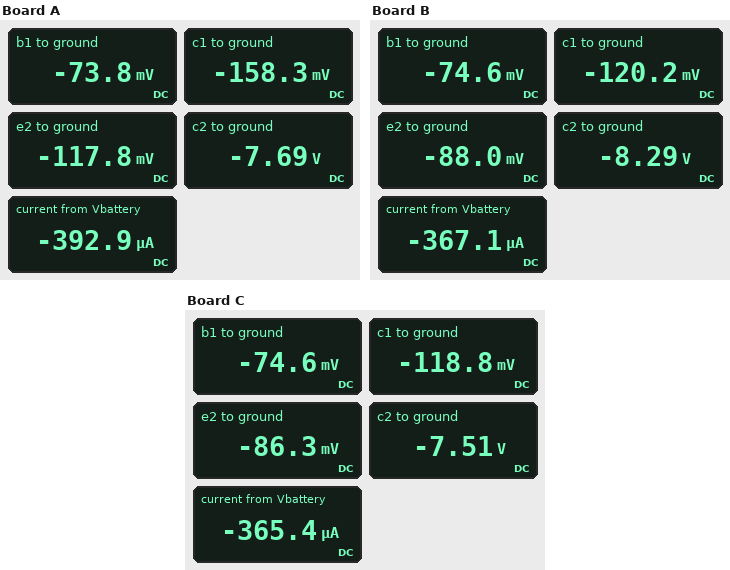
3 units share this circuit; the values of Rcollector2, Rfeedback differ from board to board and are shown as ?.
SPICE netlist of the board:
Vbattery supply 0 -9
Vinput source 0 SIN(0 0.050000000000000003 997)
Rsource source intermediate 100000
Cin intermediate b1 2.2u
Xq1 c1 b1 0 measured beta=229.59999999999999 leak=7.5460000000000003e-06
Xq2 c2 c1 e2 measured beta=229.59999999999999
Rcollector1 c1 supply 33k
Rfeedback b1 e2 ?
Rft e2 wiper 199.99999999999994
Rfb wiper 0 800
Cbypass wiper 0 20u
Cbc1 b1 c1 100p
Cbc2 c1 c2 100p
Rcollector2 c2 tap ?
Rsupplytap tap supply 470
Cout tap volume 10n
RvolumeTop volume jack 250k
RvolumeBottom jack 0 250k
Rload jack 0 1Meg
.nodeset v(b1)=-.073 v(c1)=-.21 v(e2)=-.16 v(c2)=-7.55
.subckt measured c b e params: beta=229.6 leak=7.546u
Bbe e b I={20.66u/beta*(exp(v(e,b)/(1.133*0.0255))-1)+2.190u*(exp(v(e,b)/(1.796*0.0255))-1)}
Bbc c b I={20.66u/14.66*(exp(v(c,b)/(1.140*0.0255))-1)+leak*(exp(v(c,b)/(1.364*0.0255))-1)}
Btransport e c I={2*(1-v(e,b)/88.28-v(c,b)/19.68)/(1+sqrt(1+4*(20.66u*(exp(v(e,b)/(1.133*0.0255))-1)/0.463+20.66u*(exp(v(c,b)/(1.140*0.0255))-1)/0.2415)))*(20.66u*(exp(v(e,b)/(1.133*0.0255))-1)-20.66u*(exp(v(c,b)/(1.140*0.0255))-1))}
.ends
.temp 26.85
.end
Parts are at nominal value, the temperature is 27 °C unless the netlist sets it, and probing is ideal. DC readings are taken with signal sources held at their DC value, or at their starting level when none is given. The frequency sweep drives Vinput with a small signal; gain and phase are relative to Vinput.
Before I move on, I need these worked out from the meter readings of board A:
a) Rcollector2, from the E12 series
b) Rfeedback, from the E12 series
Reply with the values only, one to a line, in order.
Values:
10 kΩ
27 kΩ
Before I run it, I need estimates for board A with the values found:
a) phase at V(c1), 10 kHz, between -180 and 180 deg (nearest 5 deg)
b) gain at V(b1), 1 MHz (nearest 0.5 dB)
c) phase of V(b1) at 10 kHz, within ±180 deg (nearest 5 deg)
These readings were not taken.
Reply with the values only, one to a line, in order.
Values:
165 deg
-49.5 dB
25 deg
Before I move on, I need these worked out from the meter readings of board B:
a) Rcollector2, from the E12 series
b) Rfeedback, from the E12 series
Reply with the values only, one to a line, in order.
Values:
6.8 kΩ
3.9 kΩ
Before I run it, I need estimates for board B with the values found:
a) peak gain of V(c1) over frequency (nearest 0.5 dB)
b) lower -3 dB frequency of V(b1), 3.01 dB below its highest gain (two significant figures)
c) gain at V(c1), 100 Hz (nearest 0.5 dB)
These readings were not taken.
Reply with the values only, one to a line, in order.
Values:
-25.5 dB
69 kHz
-25.5 dB
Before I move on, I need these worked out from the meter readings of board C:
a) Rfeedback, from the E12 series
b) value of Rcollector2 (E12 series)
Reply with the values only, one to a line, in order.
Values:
3.3 kΩ
15 kΩ
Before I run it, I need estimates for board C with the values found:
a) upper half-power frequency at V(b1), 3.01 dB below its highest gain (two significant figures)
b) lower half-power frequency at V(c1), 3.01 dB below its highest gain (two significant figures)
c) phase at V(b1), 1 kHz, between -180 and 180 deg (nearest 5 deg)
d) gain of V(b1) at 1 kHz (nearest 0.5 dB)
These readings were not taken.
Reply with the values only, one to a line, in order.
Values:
570 kHz
12 Hz
5 deg
-55.0 dB
